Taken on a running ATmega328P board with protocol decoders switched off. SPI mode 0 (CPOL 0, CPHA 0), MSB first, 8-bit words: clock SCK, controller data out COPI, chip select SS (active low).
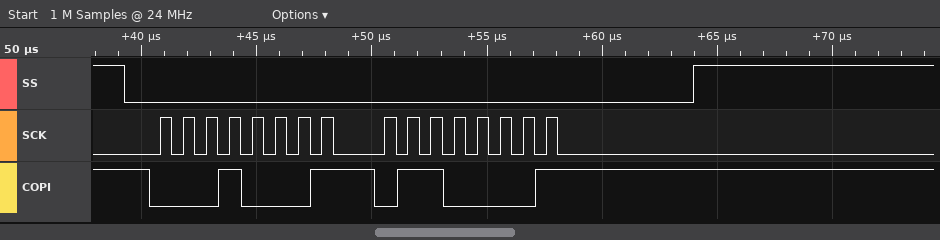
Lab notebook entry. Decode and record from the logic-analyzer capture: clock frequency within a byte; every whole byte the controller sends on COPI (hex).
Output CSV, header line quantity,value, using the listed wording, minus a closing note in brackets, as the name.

quantity,value
clock frequency within a byte,1 MHz
every whole byte the controller sends on COPI,11 61
